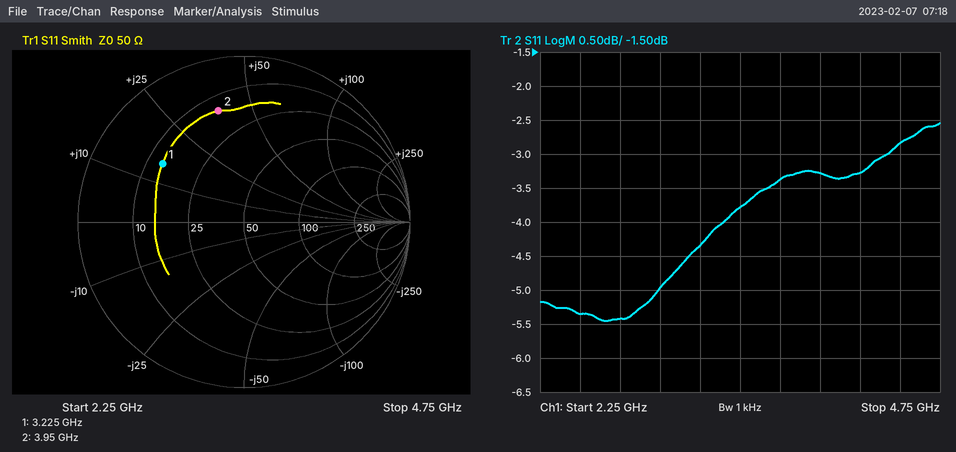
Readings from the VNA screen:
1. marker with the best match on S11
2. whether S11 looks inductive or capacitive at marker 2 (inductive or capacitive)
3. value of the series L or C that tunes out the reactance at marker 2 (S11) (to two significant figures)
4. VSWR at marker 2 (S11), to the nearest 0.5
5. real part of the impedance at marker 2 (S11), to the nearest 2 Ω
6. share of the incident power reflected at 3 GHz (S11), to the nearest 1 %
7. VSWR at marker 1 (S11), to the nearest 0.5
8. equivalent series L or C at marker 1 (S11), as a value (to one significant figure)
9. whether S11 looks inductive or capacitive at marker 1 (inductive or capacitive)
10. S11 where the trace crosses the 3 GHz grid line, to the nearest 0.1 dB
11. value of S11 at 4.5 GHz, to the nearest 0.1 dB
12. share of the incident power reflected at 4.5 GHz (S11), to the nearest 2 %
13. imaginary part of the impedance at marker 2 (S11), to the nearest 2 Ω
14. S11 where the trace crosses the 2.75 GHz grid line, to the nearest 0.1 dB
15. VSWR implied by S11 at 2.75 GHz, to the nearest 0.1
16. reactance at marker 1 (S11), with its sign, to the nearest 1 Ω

marker 1
inductive
1.1 pF
5.5
14 Ω
32 %
4.0
700 pH
inductive
-5.0 dB
-2.8 dB
52 %
+38 Ω
-5.4 dB
3.3
+15 Ω
